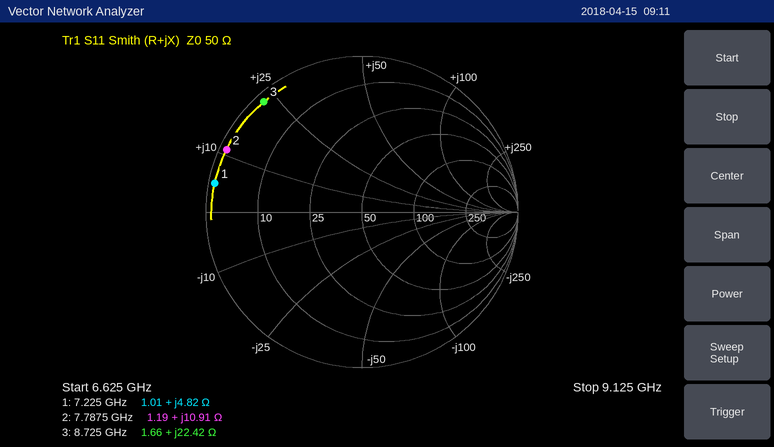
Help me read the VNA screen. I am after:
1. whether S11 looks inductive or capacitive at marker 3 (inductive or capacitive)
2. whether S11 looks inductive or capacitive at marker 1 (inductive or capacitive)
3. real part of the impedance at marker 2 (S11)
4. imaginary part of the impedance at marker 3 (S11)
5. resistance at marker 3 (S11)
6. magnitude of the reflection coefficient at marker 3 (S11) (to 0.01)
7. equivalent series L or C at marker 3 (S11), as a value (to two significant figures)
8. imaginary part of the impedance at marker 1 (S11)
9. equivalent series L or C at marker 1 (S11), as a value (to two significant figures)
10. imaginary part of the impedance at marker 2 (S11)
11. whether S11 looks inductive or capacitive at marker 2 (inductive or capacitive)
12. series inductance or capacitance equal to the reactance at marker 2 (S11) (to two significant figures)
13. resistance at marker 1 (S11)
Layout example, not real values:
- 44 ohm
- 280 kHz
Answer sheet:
- inductive
- inductive
- 1.19 Ω
- +22.42 Ω
- 1.66 Ω
- 0.95
- 410 pH
- +4.82 Ω
- 110 pH
- +10.91 Ω
- inductive
- 220 pH
- 1.01 Ω
